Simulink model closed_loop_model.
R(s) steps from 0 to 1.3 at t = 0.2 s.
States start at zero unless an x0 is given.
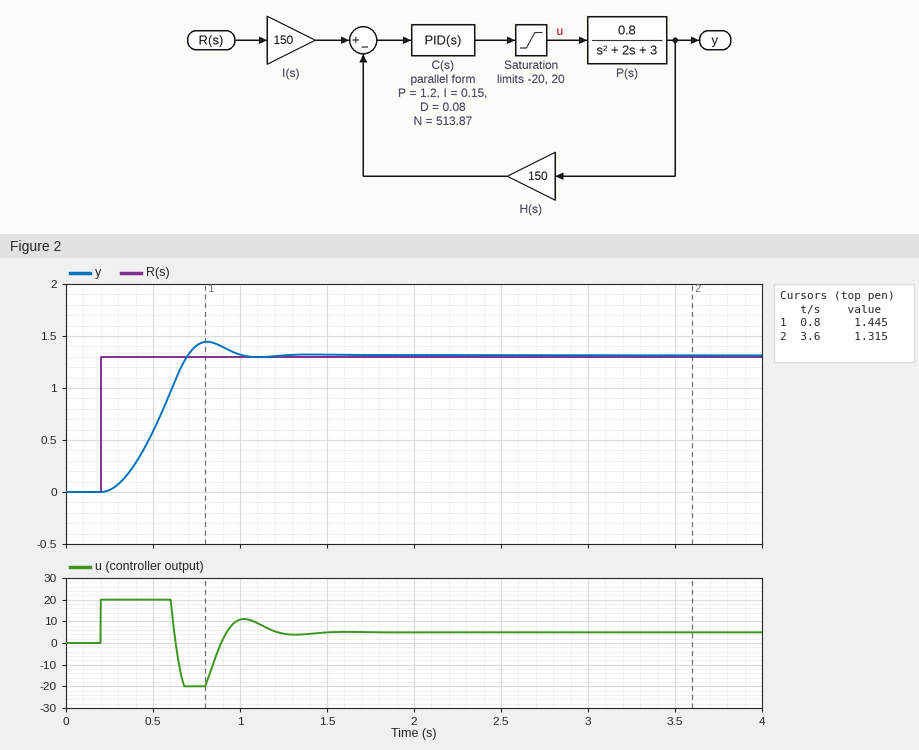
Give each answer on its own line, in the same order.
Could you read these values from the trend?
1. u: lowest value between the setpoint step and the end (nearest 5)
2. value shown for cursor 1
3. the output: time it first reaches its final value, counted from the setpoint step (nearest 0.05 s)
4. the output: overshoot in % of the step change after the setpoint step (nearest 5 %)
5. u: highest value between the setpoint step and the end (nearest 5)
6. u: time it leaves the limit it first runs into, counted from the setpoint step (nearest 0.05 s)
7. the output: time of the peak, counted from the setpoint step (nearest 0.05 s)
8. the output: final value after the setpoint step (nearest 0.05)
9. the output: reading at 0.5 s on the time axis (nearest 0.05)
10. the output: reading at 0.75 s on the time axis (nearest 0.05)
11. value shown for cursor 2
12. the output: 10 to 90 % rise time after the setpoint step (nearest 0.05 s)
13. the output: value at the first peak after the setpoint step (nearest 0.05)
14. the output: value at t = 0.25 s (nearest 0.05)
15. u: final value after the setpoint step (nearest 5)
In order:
-20
1.445
0.50 s
10 %
20
0.40 s
0.60 s
1.30
0.60
1.40
1.315
0.30 s
1.45
0.00
5
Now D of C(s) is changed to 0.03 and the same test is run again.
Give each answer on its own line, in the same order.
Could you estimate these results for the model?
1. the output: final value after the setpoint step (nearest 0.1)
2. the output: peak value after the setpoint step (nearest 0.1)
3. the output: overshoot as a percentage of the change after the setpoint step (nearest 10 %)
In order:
1.3
1.6
20 %
